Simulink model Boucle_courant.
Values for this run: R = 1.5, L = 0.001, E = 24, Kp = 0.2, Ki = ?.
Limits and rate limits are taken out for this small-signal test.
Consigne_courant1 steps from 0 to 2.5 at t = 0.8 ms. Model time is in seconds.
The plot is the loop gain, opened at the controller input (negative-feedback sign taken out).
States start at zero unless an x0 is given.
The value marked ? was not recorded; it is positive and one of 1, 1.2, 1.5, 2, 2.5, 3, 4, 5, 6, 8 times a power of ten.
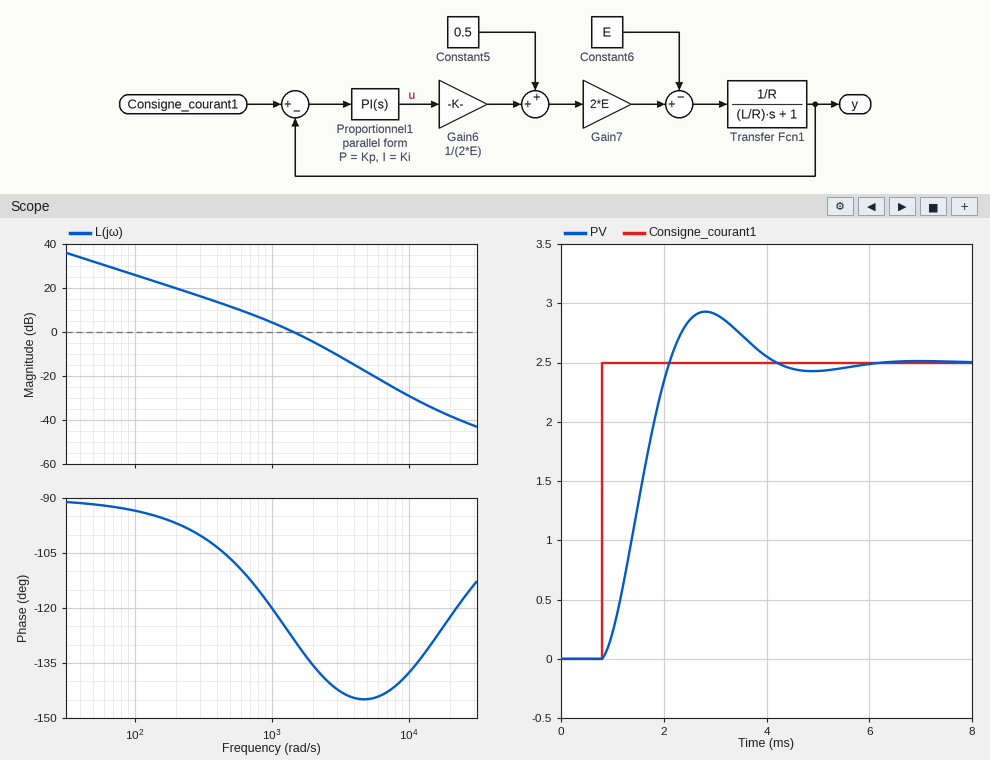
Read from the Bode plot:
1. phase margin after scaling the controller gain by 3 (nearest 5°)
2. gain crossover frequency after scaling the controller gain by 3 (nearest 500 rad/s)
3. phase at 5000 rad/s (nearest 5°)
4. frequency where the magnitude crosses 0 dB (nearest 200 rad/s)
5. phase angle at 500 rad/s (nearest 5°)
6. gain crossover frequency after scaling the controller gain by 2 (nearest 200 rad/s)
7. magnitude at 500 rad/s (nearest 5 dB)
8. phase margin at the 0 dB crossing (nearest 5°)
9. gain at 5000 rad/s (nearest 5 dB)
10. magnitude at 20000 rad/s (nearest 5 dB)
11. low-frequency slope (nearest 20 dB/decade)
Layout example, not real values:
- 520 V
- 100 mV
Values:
- 40°
- 3000 rad/s
- -145°
- 1400 rad/s
- -105°
- 2200 rad/s
- 10 dB
- 50°
- -20 dB
- -40 dB
- -20 dB/decade
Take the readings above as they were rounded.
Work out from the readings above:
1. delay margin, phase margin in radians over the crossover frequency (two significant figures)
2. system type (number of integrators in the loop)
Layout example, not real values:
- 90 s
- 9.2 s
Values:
- 0.00062 s
- 1
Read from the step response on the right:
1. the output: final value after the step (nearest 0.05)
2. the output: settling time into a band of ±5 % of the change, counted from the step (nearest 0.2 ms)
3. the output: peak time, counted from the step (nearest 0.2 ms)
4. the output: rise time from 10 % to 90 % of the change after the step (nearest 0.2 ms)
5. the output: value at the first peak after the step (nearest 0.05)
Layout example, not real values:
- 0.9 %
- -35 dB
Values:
- 2.50
- 3.0 ms
- 2.0 ms
- 1.0 ms
- 2.95
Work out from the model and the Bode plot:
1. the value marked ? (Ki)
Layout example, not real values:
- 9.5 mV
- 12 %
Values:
- 3000
